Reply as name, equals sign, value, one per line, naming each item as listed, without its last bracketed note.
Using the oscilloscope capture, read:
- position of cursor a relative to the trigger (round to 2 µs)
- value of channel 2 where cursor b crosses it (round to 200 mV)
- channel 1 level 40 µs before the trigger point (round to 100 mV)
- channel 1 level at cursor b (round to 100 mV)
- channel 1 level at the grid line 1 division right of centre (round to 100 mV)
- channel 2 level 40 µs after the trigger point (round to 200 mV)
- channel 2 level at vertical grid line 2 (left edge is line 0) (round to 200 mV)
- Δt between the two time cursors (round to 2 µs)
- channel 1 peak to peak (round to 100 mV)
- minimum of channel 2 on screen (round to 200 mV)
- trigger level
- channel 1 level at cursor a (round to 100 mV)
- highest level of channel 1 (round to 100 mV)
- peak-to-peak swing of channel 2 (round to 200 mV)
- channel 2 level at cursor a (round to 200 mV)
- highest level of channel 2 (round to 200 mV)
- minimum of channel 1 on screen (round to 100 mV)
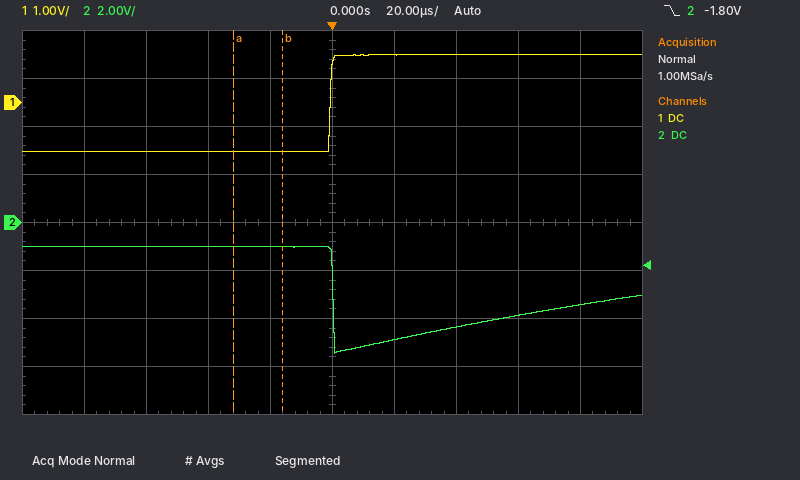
position of cursor a relative to the trigger = -32 µs
value of channel 2 where cursor b crosses it = -1.0 V
channel 1 level 40 µs before the trigger point = -1.0 V
channel 1 level at cursor b = -1.0 V
channel 1 level at the grid line 1 division right of centre = 1.0 V
channel 2 level 40 µs after the trigger point = -4.4 V
channel 2 level at vertical grid line 2 (left edge is line 0) = -1.0 V
Δt between the two time cursors = 16 µs
channel 1 peak to peak = 2.0 V
minimum of channel 2 on screen = -5.4 V
trigger level = -1.80 V
channel 1 level at cursor a = -1.0 V
highest level of channel 1 = 1.0 V
peak-to-peak swing of channel 2 = 4.4 V
channel 2 level at cursor a = -1.0 V
highest level of channel 2 = -1.0 V
minimum of channel 1 on screen = -1.0 V
